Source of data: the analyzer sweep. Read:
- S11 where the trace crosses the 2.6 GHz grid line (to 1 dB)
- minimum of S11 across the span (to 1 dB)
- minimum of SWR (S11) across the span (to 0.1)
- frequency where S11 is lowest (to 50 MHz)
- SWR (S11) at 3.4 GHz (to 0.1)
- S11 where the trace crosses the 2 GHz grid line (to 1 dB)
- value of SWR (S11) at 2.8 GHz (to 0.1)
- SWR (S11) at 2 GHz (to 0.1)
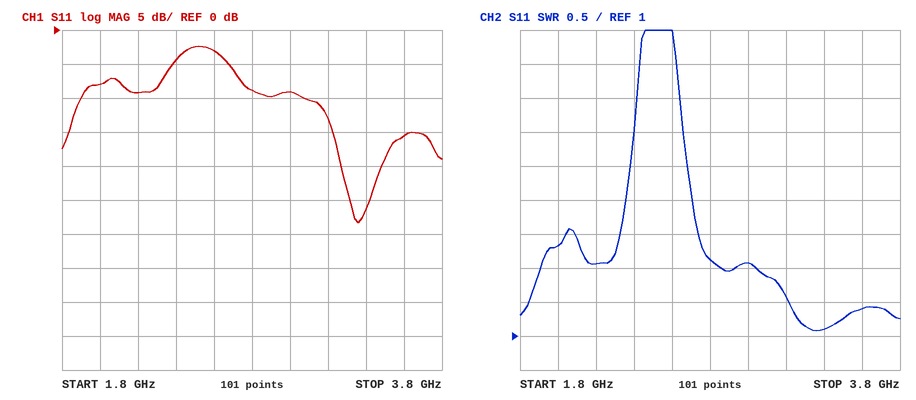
-3 dB
-28 dB
1.1
3.35 GHz
1.1
-8 dB
2.1
2.3
